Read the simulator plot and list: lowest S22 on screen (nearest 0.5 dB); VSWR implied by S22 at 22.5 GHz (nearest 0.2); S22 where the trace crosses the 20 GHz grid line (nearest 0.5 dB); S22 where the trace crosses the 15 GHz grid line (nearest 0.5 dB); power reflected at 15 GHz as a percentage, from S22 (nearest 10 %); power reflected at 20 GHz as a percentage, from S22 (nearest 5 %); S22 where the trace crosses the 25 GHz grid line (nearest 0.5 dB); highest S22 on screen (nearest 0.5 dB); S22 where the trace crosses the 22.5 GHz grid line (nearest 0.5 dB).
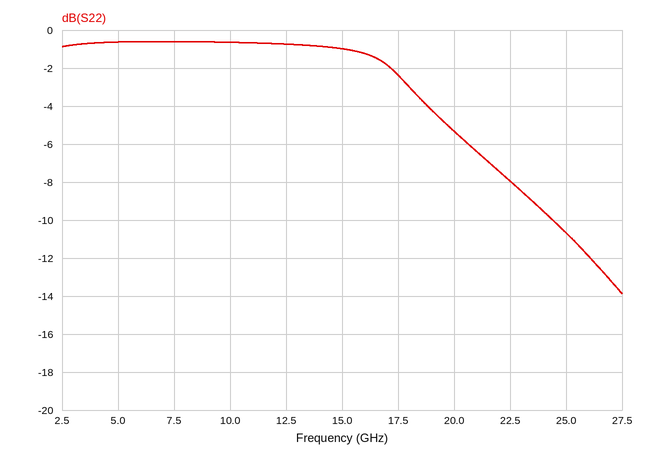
-14.0 dB
2.4
-5.5 dB
-1.0 dB
80 %
30 %
-10.5 dB
-0.5 dB
-8.0 dB
